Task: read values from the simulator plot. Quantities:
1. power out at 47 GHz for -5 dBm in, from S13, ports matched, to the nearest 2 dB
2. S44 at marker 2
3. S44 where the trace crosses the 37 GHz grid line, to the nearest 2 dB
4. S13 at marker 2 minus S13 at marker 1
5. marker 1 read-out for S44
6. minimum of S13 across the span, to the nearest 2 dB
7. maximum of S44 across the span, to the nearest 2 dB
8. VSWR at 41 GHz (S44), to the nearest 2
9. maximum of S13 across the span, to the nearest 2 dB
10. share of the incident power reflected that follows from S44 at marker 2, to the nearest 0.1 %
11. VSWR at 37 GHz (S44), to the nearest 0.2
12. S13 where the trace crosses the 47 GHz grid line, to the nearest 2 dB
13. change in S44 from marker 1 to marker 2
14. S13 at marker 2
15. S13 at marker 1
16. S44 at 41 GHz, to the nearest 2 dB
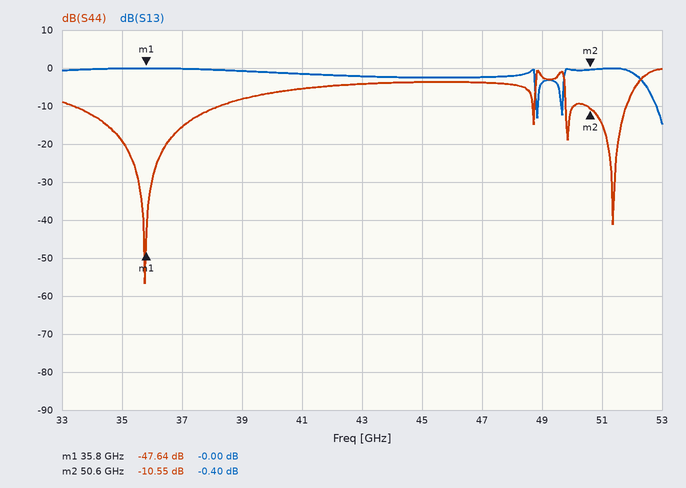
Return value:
-8 dBm
-10.55 dB
-16 dB
-0.40 dB
-47.64 dB
-14 dB
0 dB
4
0 dB
8.8 %
1.4
-2 dB
37.09 dB
-0.40 dB
-0.00 dB
-6 dB
